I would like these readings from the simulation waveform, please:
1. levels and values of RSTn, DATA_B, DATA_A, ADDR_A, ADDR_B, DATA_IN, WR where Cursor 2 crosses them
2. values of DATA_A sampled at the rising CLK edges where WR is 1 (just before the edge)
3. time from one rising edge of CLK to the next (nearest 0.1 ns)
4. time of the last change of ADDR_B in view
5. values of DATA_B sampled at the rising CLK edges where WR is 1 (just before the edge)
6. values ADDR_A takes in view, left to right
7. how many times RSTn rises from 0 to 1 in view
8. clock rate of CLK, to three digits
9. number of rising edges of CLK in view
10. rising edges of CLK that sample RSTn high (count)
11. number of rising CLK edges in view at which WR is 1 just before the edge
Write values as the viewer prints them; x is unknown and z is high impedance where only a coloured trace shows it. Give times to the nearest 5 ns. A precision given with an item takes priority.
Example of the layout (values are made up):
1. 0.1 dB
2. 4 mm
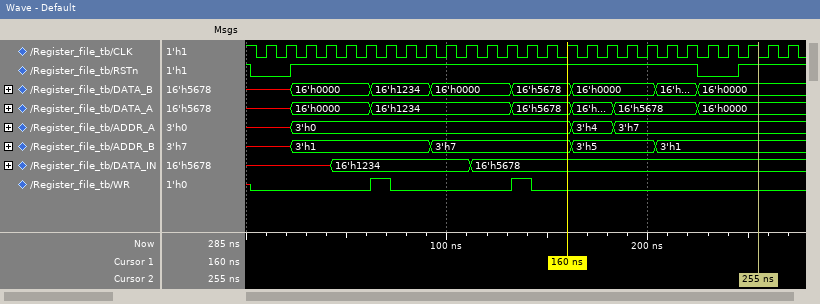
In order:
1. RSTn=1, DATA_B=16'h0000, DATA_A=16'h0000, ADDR_A=3'h7, ADDR_B=3'h1, DATA_IN=16'h5678, WR=0
2. 16'h1234, 16'h5678
3. 10 ns
4. 205 ns
5. 16'h1234, 16'h5678
6. x, 3'h0, 3'h4, 3'h7
7. 2
8. 100 MHz
9. 27
10. 23
11. 2
